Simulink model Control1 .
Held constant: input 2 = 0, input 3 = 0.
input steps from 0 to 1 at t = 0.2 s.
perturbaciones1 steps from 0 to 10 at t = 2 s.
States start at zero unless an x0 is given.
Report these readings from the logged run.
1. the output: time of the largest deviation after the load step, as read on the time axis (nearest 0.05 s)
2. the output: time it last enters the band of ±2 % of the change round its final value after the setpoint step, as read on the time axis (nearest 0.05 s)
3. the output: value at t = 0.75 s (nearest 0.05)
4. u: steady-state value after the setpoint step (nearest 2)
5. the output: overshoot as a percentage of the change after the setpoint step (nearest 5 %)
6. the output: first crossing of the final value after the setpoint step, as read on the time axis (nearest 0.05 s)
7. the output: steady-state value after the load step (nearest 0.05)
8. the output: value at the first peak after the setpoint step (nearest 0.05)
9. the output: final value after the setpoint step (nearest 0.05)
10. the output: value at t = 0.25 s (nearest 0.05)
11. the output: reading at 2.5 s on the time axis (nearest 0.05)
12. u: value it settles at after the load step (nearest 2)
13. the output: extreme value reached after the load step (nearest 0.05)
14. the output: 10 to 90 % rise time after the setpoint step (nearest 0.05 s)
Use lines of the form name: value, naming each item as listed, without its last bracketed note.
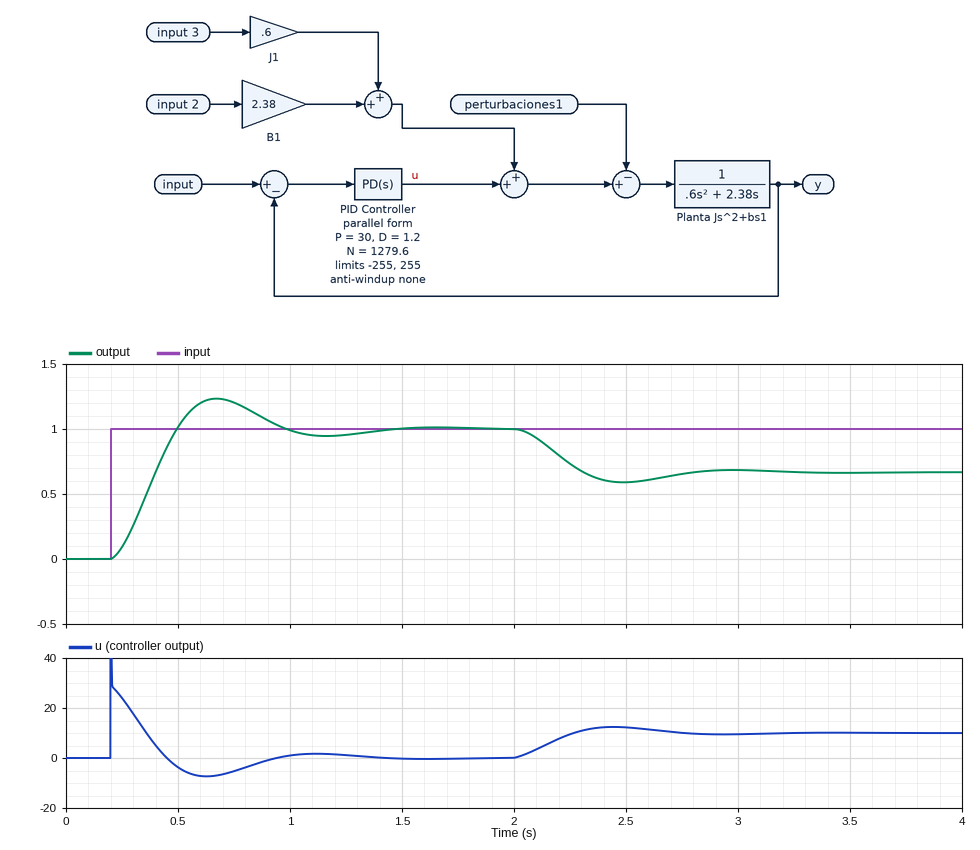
the output: time of the largest deviation after the load step, as read on the time axis: 2.50 s
the output: time it last enters the band of ±2 % of the change round its final value after the setpoint step, as read on the time axis: 1.35 s
the output: value at t = 0.75 s: 1.20
u: steady-state value after the setpoint step: 0
the output: overshoot as a percentage of the change after the setpoint step: 25 %
the output: first crossing of the final value after the setpoint step, as read on the time axis: 0.50 s
the output: steady-state value after the load step: 0.65
the output: value at the first peak after the setpoint step: 1.25
the output: final value after the setpoint step: 1.00
the output: value at t = 0.25 s: 0.10
the output: reading at 2.5 s on the time axis: 0.60
u: value it settles at after the load step: 10
the output: extreme value reached after the load step: 0.60
the output: 10 to 90 % rise time after the setpoint step: 0.20 s
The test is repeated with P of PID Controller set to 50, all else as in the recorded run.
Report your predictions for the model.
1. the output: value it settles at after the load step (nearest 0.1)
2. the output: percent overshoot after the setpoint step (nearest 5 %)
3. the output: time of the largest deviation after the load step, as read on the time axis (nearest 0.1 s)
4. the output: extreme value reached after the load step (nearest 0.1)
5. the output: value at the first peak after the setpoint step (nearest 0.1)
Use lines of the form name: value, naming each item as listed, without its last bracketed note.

the output: value it settles at after the load step: 0.8
the output: percent overshoot after the setpoint step: 35 %
the output: time of the largest deviation after the load step, as read on the time axis: 2.4 s
the output: extreme value reached after the load step: 0.7
the output: value at the first peak after the setpoint step: 1.3
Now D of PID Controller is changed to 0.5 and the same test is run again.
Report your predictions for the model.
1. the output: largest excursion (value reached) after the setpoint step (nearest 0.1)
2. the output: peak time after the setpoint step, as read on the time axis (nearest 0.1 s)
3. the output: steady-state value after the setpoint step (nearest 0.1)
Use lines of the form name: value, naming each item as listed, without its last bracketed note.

the output: largest excursion (value reached) after the setpoint step: 1.3
the output: peak time after the setpoint step, as read on the time axis: 0.7 s
the output: steady-state value after the setpoint step: 1.0
